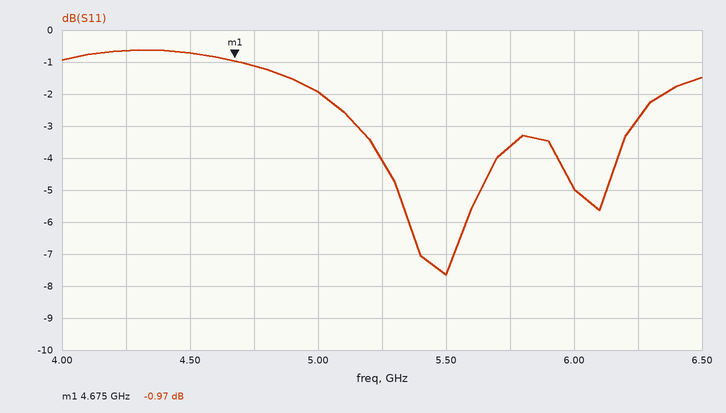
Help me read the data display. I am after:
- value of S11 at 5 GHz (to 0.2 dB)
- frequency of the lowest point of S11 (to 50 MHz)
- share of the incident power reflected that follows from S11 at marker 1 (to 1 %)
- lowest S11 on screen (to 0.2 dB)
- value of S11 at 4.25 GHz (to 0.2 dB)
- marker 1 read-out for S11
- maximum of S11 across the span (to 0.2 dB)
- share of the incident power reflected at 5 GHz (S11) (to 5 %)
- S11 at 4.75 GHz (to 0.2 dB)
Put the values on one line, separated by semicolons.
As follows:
-2.0 dB; 5.50 GHz; 80 %; -7.6 dB; -0.6 dB; -0.97 dB; -0.6 dB; 65 %; -1.2 dB
